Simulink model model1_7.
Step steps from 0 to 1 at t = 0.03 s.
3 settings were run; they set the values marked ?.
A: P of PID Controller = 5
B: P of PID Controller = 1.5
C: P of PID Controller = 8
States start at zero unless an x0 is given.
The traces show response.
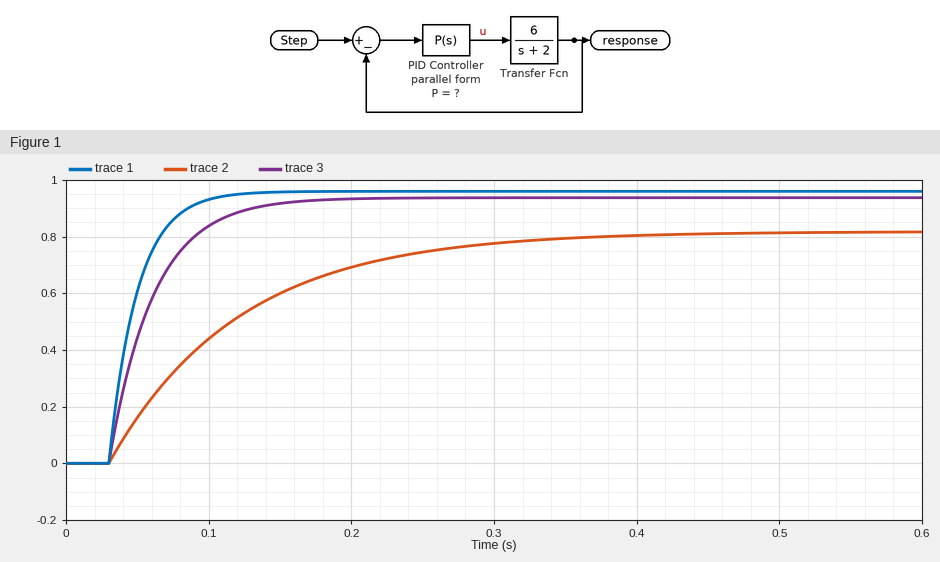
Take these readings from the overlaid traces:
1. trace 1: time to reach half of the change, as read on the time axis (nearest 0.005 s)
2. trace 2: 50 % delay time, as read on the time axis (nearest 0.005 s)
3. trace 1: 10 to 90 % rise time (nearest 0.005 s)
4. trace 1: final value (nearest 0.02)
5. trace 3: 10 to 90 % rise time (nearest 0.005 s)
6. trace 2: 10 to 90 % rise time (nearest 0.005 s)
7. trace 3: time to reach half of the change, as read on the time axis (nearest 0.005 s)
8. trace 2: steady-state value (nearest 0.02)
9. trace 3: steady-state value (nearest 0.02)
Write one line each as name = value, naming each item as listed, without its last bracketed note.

trace 1: time to reach half of the change, as read on the time axis = 0.045 s
trace 2: 50 % delay time, as read on the time axis = 0.095 s
trace 1: 10 to 90 % rise time = 0.045 s
trace 1: final value = 0.96
trace 3: 10 to 90 % rise time = 0.070 s
trace 2: 10 to 90 % rise time = 0.200 s
trace 3: time to reach half of the change, as read on the time axis = 0.050 s
trace 2: steady-state value = 0.82
trace 3: steady-state value = 0.94
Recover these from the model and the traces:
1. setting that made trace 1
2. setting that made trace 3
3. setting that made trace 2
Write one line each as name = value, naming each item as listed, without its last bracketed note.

setting that made trace 1 = C
setting that made trace 3 = A
setting that made trace 2 = B
